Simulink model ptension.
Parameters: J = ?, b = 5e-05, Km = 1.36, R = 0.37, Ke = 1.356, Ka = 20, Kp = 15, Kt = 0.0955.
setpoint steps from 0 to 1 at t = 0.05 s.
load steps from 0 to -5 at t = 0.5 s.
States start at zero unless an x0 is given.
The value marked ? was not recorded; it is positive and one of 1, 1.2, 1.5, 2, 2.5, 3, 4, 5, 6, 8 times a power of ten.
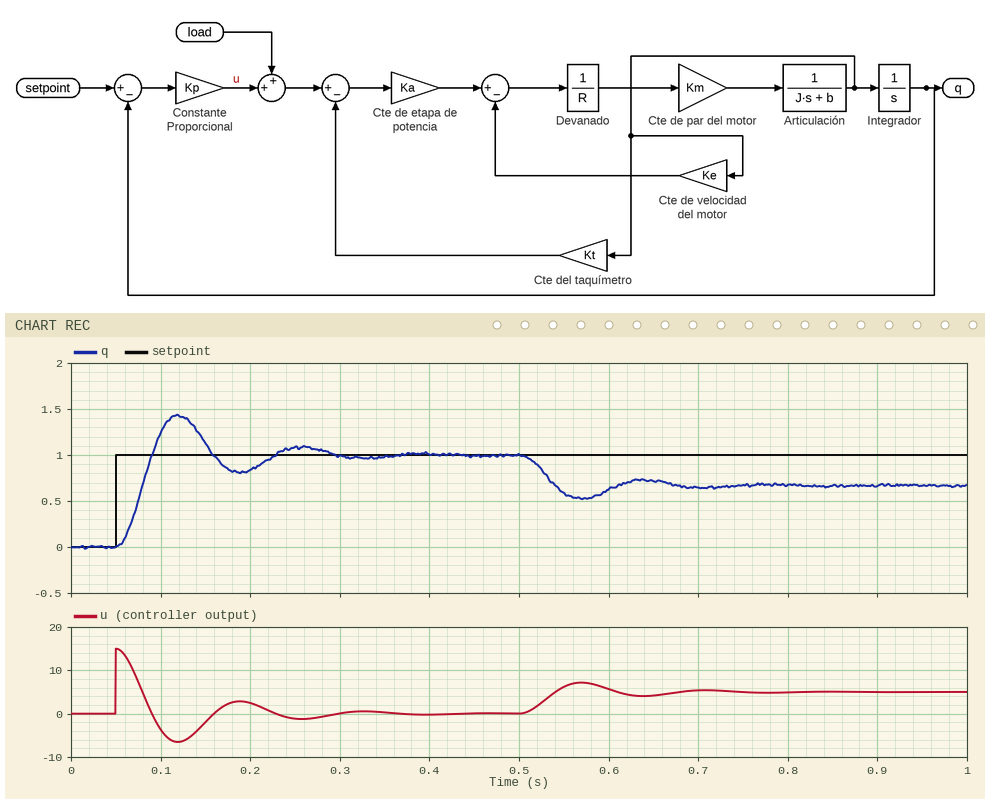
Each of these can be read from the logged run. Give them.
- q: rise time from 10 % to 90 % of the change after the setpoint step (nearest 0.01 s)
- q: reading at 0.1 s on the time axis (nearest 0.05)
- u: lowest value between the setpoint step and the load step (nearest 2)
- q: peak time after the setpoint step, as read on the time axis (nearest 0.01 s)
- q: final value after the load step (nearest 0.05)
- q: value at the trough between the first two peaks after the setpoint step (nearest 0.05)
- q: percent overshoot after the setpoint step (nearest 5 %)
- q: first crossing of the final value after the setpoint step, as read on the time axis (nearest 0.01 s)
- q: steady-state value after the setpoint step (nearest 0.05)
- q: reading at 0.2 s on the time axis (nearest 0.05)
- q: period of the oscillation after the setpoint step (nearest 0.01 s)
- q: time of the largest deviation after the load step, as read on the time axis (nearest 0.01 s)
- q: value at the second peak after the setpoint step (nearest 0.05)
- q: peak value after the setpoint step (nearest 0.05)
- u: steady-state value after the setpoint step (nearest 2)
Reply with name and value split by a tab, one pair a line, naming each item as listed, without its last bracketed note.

q: rise time from 10 % to 90 % of the change after the setpoint step	0.03 s
q: reading at 0.1 s on the time axis	1.25
u: lowest value between the setpoint step and the load step	-6
q: peak time after the setpoint step, as read on the time axis	0.12 s
q: final value after the load step	0.65
q: value at the trough between the first two peaks after the setpoint step	0.80
q: percent overshoot after the setpoint step	45 %
q: first crossing of the final value after the setpoint step, as read on the time axis	0.09 s
q: steady-state value after the setpoint step	1.00
q: reading at 0.2 s on the time axis	0.85
q: period of the oscillation after the setpoint step	0.14 s
q: time of the largest deviation after the load step, as read on the time axis	0.57 s
q: value at the second peak after the setpoint step	1.10
q: peak value after the setpoint step	1.45
u: steady-state value after the setpoint step	0
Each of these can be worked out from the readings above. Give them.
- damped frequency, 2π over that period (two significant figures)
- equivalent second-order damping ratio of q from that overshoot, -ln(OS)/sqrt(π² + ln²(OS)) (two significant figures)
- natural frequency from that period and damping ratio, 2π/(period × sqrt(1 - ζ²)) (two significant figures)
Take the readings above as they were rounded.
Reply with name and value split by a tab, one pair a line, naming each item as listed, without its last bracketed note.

damped frequency, 2π over that period	45 rad/s
equivalent second-order damping ratio of q from that overshoot, -ln(OS)/sqrt(π² + ln²(OS))	0.25
natural frequency from that period and damping ratio, 2π/(period × sqrt(1 - ζ²))	46 rad/s
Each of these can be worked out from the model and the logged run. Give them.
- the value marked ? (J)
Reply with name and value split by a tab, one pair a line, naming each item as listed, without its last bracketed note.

the value marked ?	0.5
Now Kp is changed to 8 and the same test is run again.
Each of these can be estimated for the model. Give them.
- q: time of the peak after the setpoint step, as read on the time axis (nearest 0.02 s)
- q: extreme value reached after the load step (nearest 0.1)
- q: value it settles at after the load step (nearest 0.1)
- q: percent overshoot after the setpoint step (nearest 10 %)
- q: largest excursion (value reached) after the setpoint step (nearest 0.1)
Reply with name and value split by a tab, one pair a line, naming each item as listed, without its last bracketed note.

q: time of the peak after the setpoint step, as read on the time axis	0.14 s
q: extreme value reached after the load step	0.2
q: value it settles at after the load step	0.4
q: percent overshoot after the setpoint step	30 %
q: largest excursion (value reached) after the setpoint step	1.3
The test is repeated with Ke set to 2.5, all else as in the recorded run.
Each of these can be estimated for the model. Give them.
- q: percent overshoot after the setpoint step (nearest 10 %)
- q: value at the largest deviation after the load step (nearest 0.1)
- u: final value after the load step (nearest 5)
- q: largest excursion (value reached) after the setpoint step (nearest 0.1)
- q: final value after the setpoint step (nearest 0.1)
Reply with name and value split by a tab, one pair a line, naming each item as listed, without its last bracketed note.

q: percent overshoot after the setpoint step	30 %
q: value at the largest deviation after the load step	0.6
u: final value after the load step	5
q: largest excursion (value reached) after the setpoint step	1.3
q: final value after the setpoint step	1.0
